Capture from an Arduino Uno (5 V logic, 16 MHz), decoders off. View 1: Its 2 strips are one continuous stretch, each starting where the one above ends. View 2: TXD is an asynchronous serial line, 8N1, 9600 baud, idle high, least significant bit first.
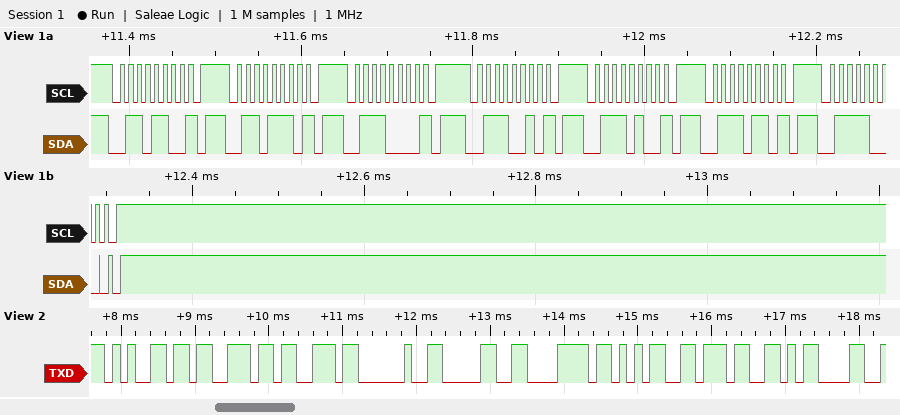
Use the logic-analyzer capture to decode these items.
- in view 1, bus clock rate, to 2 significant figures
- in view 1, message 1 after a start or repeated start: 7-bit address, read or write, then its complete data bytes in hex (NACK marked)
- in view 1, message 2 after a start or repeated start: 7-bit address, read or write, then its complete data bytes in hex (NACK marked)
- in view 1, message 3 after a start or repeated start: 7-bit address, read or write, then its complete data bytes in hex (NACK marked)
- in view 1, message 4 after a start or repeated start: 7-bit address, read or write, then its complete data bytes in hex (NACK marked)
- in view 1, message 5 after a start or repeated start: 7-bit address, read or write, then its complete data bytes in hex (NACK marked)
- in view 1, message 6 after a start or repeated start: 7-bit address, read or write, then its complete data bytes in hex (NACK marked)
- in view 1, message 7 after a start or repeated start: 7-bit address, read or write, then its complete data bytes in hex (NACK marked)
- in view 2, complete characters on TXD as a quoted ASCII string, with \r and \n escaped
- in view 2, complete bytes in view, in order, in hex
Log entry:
100 kHz
0x36 write NACK
0x37 write NACK
0x38 write NACK
0x39 write NACK
0x3A write NACK
0x3B write NACK
0x3C write
"ess 0x57\r"
65 73 73 20 30 78 35 37 0D
